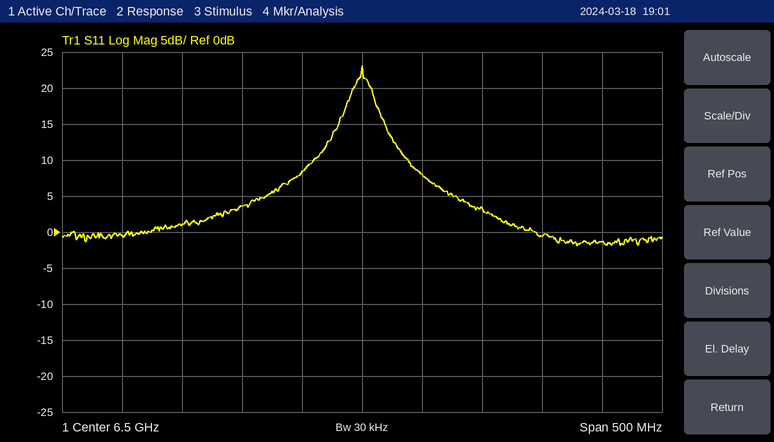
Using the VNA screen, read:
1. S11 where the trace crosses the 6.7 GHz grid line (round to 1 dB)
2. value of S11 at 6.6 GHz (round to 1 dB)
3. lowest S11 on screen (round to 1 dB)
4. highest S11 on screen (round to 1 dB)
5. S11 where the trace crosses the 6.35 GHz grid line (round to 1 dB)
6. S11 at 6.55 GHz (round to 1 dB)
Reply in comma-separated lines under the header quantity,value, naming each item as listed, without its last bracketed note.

quantity,value
S11 where the trace crosses the 6.7 GHz grid line,-1 dB
value of S11 at 6.6 GHz,3 dB
lowest S11 on screen,-2 dB
highest S11 on screen,23 dB
S11 where the trace crosses the 6.35 GHz grid line,1 dB
S11 at 6.55 GHz,8 dB
